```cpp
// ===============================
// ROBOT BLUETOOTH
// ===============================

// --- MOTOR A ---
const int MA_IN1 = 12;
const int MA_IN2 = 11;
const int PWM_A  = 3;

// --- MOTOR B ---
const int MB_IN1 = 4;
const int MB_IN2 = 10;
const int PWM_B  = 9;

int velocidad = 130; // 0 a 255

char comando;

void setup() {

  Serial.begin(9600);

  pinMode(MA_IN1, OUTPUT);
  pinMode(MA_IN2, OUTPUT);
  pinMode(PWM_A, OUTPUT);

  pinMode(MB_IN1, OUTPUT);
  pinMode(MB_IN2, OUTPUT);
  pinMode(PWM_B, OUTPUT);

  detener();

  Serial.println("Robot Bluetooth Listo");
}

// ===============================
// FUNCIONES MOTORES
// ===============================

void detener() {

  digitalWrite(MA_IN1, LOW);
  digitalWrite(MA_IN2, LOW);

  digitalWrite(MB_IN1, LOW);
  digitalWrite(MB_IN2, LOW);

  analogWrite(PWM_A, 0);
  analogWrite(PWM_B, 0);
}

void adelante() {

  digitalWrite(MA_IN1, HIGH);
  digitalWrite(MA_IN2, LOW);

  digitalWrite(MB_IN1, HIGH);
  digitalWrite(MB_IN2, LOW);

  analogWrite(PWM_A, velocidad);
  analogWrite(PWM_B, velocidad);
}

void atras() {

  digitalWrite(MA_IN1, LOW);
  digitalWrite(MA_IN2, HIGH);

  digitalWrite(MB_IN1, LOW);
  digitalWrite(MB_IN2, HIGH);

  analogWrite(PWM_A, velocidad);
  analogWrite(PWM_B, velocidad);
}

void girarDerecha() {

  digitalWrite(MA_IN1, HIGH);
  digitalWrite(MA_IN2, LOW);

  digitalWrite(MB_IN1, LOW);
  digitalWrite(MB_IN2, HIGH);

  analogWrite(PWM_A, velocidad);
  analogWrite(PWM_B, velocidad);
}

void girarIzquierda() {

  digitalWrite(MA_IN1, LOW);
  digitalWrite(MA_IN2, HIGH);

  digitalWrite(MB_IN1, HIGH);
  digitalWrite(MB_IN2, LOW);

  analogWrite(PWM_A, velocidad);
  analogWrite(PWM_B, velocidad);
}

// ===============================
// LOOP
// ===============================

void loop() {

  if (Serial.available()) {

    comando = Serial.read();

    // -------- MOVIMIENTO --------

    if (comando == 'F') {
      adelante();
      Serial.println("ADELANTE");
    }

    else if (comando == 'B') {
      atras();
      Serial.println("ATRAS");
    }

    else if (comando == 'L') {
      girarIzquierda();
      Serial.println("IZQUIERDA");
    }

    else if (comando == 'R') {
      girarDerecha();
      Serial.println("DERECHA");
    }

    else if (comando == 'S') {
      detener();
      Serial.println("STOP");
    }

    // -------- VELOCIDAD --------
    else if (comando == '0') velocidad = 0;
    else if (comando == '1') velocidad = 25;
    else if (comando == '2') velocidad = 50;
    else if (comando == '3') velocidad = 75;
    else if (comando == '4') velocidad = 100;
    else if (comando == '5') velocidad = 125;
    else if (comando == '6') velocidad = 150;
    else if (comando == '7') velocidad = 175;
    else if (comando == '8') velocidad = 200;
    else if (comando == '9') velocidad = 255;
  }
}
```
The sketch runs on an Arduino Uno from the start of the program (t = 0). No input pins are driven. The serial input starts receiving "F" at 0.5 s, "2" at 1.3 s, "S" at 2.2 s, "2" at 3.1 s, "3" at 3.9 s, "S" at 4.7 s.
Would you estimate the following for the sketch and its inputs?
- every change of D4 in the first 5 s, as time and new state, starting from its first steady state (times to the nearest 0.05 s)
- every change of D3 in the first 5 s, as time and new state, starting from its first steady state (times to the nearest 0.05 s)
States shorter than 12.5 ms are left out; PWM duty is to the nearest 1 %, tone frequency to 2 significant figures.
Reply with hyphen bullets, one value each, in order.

- 0 s low; 0.5 s high; 2.2 s low
- 0 s low; 0.5 s PWM 51 %; 2.2 s low
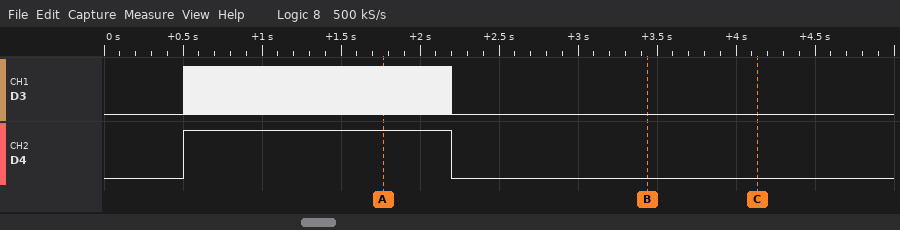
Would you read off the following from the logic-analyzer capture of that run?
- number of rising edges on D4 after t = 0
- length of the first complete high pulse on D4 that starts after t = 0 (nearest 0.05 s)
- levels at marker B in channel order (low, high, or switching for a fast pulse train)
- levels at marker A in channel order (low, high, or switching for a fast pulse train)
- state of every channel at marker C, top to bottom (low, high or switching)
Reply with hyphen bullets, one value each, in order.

- 1
- 1.70 s
- D3 low, D4 low
- D3 switching, D4 high
- D3 low, D4 low
